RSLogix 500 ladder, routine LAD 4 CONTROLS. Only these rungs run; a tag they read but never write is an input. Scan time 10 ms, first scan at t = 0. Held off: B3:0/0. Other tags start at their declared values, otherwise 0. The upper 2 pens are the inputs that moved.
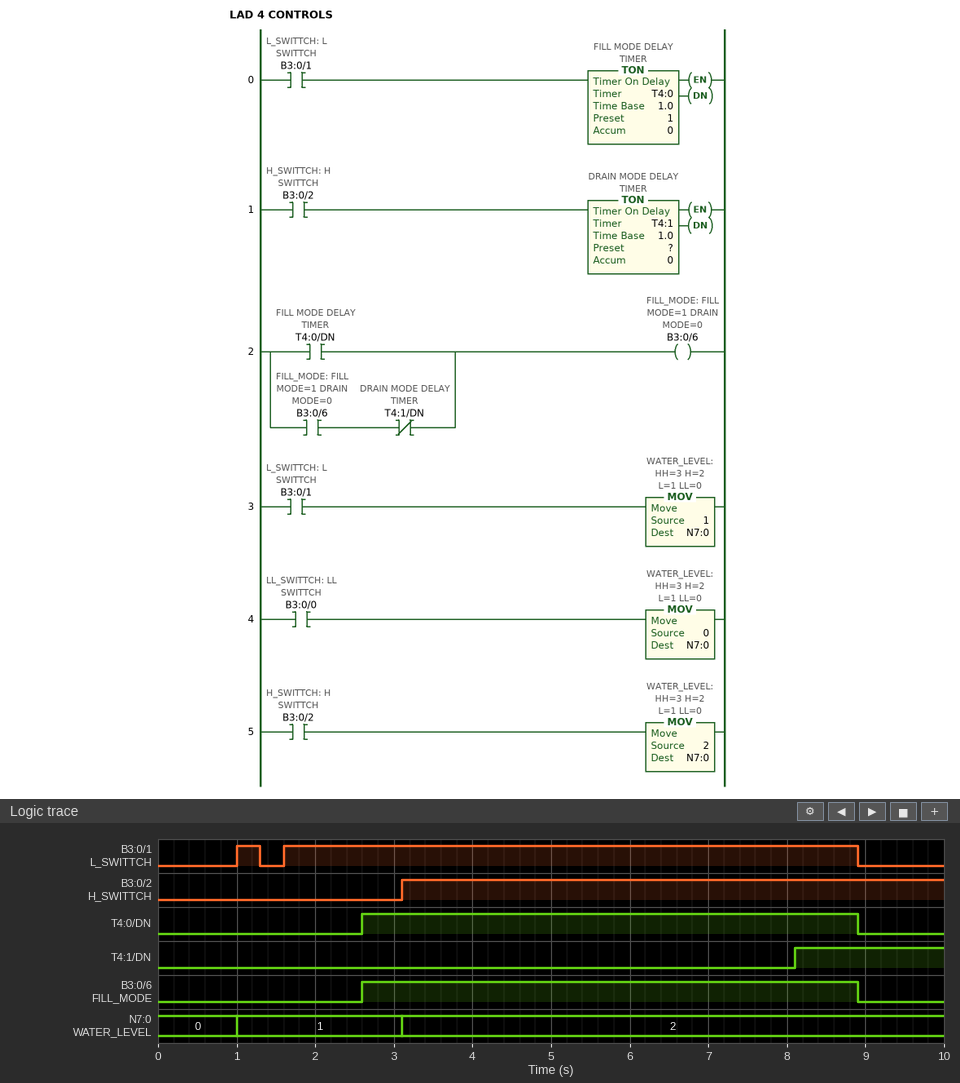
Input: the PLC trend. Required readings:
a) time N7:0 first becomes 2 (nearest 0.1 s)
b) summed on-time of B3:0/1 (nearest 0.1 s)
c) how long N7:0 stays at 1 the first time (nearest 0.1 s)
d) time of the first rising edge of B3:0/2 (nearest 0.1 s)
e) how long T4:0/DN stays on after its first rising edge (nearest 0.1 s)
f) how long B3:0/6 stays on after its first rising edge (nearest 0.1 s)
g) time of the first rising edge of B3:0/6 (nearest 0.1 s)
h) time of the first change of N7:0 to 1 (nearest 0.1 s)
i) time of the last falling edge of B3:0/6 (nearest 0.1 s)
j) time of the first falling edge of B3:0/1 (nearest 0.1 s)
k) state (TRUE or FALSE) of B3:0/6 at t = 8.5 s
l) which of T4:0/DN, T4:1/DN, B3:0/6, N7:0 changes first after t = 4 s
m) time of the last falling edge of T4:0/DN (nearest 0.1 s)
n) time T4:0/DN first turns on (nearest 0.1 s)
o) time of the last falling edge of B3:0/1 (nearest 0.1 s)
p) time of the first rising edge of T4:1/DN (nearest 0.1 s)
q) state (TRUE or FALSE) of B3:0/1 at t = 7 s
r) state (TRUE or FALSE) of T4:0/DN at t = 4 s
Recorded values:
3.1 s
7.6 s
2.1 s
3.1 s
6.3 s
6.3 s
2.6 s
1.0 s
8.9 s
1.3 s
TRUE
T4:1/DN
8.9 s
2.6 s
8.9 s
8.1 s
TRUE
TRUE
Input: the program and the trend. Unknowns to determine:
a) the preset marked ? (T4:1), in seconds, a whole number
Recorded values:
5 s
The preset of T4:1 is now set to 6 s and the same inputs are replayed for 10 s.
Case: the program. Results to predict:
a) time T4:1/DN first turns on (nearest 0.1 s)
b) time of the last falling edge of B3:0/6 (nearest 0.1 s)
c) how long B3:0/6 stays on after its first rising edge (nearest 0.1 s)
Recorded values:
9.1 s
9.1 s
6.5 s
